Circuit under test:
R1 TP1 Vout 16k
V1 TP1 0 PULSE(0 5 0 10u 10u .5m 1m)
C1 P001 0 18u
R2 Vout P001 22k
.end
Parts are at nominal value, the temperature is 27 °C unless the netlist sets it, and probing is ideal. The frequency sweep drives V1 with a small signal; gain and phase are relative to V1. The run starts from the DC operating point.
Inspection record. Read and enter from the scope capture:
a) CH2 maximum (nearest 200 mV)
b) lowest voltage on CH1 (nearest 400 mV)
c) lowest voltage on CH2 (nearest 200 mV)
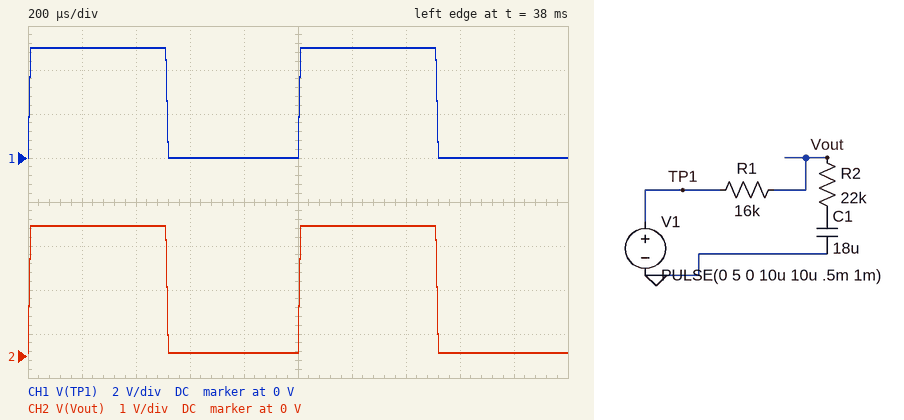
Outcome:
3.0 V
0 V
0 V
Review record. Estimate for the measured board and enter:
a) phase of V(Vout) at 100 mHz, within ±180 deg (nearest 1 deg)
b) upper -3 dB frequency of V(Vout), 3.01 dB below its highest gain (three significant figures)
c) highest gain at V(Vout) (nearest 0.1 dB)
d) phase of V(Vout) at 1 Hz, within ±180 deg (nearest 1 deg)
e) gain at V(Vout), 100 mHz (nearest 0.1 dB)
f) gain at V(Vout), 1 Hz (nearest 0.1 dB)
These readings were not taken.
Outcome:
-9 deg
405 mHz
0 dB
-9 deg
-0.5 dB
-4.3 dB
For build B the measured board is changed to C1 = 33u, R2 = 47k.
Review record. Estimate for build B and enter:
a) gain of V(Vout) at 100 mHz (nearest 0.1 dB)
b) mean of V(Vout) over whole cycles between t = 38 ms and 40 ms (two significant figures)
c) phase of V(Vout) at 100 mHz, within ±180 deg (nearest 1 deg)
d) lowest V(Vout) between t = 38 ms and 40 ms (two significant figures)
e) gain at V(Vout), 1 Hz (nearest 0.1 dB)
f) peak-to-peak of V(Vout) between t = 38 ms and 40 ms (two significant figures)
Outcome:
-1.4 dB
1.9 V
-8 deg
12 mV
-2.5 dB
3.7 V
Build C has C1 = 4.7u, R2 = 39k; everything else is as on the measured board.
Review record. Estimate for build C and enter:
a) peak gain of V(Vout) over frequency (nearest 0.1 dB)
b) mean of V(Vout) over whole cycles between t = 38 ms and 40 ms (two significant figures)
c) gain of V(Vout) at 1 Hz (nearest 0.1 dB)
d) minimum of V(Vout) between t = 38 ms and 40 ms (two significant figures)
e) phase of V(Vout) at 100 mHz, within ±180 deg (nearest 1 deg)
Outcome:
0 dB
1.9 V
-1.9 dB
100 mV
-3 deg
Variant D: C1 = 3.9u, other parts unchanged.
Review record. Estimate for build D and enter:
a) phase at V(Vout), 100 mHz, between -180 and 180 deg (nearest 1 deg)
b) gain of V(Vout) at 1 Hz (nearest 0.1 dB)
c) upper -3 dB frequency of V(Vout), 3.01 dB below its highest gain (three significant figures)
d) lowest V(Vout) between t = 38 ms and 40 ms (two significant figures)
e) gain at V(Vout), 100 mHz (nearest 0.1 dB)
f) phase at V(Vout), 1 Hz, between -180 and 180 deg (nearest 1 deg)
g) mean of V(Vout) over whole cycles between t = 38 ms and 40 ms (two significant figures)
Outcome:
-2 deg
-1.6 dB
1.87 Hz
240 mV
0 dB
-15 deg
1.7 V
